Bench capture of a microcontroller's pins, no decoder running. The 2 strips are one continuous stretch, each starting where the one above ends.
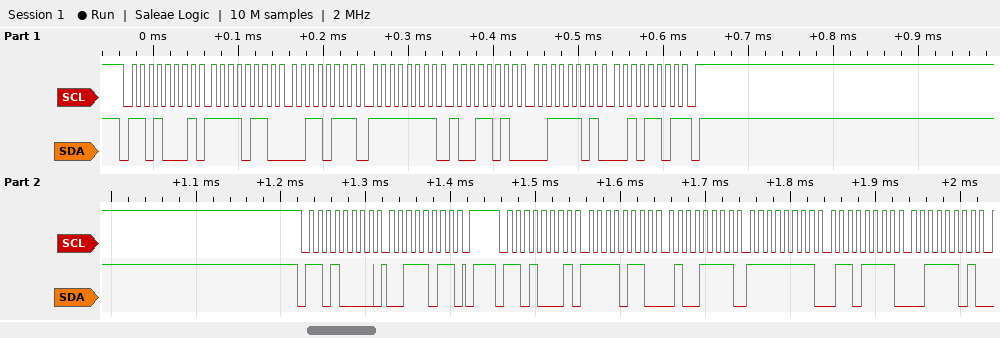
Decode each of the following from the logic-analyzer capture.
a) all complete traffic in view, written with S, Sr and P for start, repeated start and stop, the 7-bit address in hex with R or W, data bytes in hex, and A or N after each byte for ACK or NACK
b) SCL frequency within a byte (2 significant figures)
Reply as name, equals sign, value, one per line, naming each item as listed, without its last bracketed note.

all complete traffic in view, written with S, Sr and P for start, repeated start and stop, the 7-bit address in hex with R or W, data bytes in hex, and A or N after each byte for ACK or NACK = S 68R A F6 A 37 A FF A 9A A 3D A 2D N P S 68W A 3B A P S 68R A F6 A 4F A FF A 6F A 3D A
SCL frequency within a byte = 100 kHz
